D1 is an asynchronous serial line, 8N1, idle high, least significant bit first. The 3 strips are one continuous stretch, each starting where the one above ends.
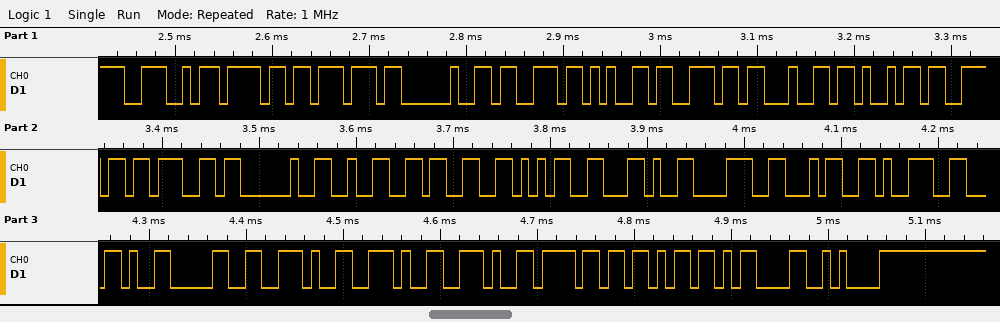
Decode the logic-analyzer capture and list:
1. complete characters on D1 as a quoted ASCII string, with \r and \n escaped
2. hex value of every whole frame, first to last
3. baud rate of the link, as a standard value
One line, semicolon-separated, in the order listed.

"Now sending 235,849,0...ok\r\n"; 4E 6F 77 20 73 65 6E 64 69 6E 67 20 32 33 35 2C 38 34 39 2C 30 2E 2E 2E 6F 6B 0D 0A; 115200 baud
